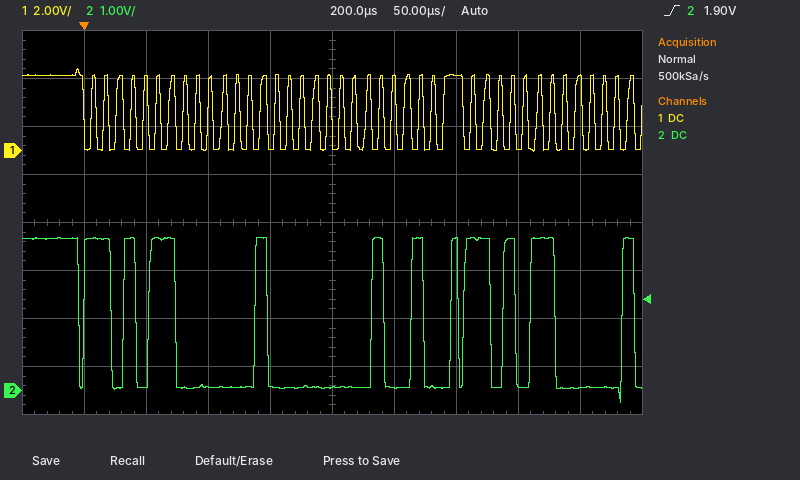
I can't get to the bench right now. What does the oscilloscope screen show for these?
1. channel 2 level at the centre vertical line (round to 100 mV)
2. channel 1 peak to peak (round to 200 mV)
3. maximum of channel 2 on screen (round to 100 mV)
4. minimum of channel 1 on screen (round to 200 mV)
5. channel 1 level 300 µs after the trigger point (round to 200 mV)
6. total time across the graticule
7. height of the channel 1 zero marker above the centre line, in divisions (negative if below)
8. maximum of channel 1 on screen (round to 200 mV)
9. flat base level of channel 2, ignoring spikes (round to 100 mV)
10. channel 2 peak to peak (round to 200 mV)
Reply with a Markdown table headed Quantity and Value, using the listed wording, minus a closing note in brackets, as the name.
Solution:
| Quantity | Value |
|---|---|
| channel 2 level at the centre vertical line | 100 mV |
| channel 1 peak to peak | 3.4 V |
| maximum of channel 2 on screen | 3.2 V |
| minimum of channel 1 on screen | 0.0 V |
| channel 1 level 300 µs after the trigger point | 3.2 V |
| total time across the graticule | 500 µs |
| height of the channel 1 zero marker above the centre line, in divisions | +1.5 div |
| maximum of channel 1 on screen | 3.4 V |
| flat base level of channel 2, ignoring spikes | 100 mV |
| channel 2 peak to peak | 3.4 V |
